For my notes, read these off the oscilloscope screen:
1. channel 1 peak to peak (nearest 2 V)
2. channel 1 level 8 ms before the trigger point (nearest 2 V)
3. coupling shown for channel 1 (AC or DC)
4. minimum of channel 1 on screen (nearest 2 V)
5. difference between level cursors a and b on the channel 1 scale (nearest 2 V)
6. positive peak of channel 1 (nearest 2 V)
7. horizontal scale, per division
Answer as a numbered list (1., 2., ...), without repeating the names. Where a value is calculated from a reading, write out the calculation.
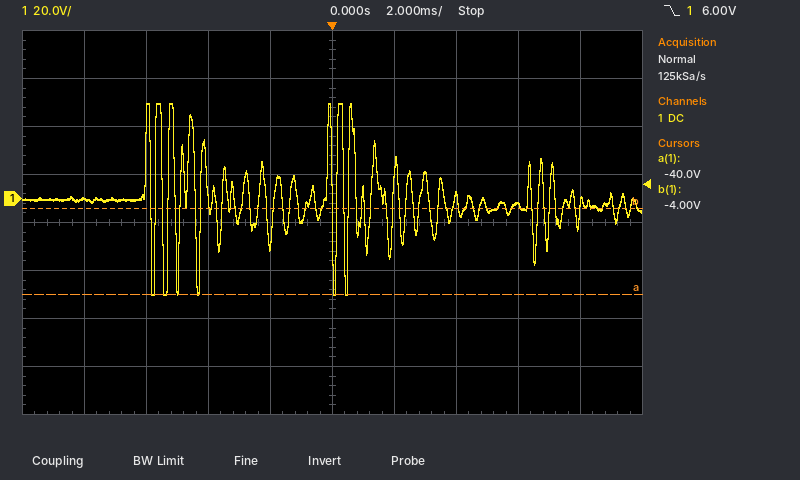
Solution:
1. 40 V − (-40 V) = 80 V
2. 0 V
3. DC
4. -40 V
5. 36 V
6. 40 V
7. 2 ms
